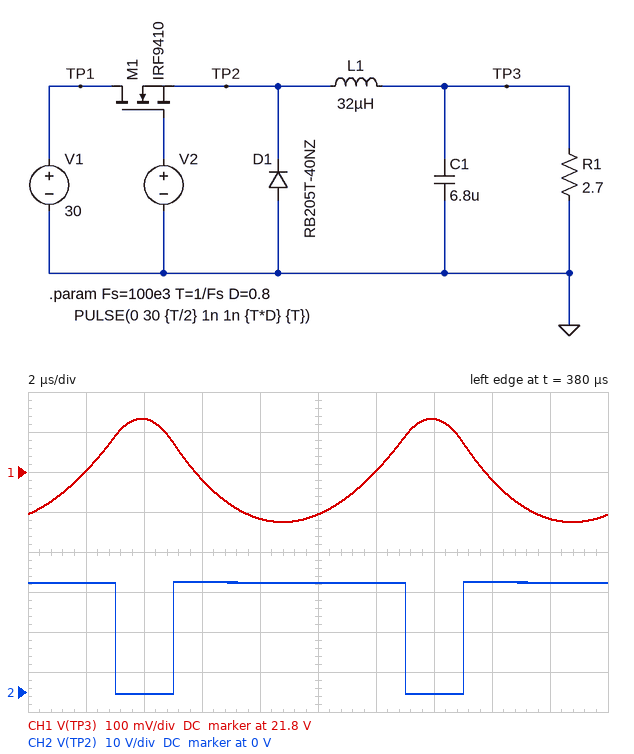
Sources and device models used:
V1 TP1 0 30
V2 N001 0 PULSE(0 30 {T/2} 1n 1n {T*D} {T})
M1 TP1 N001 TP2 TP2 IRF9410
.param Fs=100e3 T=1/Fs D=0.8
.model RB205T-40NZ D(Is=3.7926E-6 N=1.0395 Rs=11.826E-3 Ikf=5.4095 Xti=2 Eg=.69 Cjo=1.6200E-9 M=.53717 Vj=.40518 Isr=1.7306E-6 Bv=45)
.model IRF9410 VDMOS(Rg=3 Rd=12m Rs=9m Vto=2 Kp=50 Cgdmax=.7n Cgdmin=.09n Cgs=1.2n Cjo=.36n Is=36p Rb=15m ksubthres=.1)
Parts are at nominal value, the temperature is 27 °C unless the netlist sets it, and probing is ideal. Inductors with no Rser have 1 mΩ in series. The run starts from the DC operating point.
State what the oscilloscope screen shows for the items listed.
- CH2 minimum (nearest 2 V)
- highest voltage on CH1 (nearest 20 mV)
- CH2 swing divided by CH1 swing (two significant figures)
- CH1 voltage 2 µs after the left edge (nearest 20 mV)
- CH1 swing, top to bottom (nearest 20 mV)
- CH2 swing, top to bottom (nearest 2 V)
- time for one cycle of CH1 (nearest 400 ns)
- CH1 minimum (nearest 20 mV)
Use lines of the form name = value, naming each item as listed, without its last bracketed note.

CH2 minimum = 0 V
highest voltage on CH1 = 21.94 V
CH2 swing divided by CH1 swing = 110
CH1 voltage 2 µs after the left edge = 21.80 V
CH1 swing, top to bottom = 260 mV
CH2 swing, top to bottom = 28 V
time for one cycle of CH1 = 10.0 µs
CH1 minimum = 21.68 V
